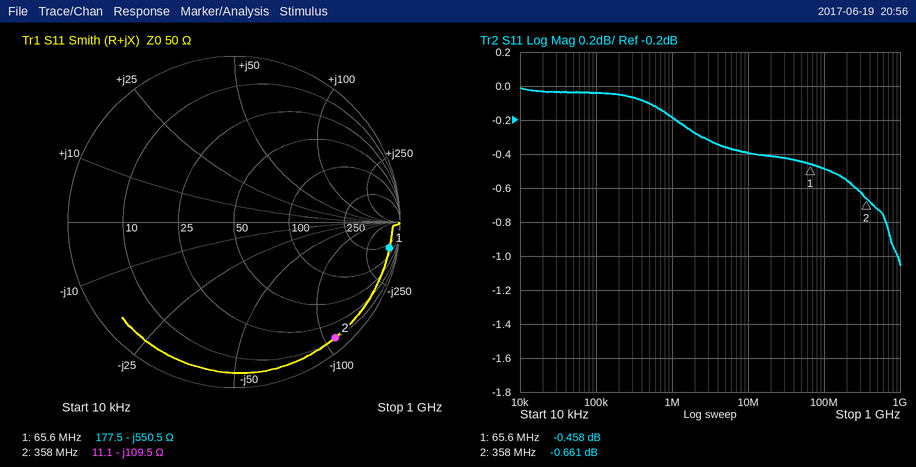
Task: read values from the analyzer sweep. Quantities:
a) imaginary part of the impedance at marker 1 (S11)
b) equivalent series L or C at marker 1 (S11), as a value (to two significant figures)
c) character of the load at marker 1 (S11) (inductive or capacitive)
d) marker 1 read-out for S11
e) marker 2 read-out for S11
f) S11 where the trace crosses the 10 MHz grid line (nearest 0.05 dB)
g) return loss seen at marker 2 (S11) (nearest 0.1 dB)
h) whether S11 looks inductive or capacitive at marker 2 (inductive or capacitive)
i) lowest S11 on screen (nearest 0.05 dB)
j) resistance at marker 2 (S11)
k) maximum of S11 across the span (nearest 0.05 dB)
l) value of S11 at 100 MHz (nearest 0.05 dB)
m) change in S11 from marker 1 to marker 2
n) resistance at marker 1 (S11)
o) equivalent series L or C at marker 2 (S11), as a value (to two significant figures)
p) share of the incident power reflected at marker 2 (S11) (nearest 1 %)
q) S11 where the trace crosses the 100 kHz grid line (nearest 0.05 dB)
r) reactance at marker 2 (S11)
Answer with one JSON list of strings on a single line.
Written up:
["-550.5 Ω", "4.4 pF", "capacitive", "-0.458 dB", "-0.661 dB", "-0.40 dB", "0.7 dB", "capacitive", "-1.05 dB", "11.1 Ω", "0.00 dB", "-0.50 dB", "-0.203 dB", "177.5 Ω", "4.1 pF", "86 %", "-0.05 dB", "-109.5 Ω"]
